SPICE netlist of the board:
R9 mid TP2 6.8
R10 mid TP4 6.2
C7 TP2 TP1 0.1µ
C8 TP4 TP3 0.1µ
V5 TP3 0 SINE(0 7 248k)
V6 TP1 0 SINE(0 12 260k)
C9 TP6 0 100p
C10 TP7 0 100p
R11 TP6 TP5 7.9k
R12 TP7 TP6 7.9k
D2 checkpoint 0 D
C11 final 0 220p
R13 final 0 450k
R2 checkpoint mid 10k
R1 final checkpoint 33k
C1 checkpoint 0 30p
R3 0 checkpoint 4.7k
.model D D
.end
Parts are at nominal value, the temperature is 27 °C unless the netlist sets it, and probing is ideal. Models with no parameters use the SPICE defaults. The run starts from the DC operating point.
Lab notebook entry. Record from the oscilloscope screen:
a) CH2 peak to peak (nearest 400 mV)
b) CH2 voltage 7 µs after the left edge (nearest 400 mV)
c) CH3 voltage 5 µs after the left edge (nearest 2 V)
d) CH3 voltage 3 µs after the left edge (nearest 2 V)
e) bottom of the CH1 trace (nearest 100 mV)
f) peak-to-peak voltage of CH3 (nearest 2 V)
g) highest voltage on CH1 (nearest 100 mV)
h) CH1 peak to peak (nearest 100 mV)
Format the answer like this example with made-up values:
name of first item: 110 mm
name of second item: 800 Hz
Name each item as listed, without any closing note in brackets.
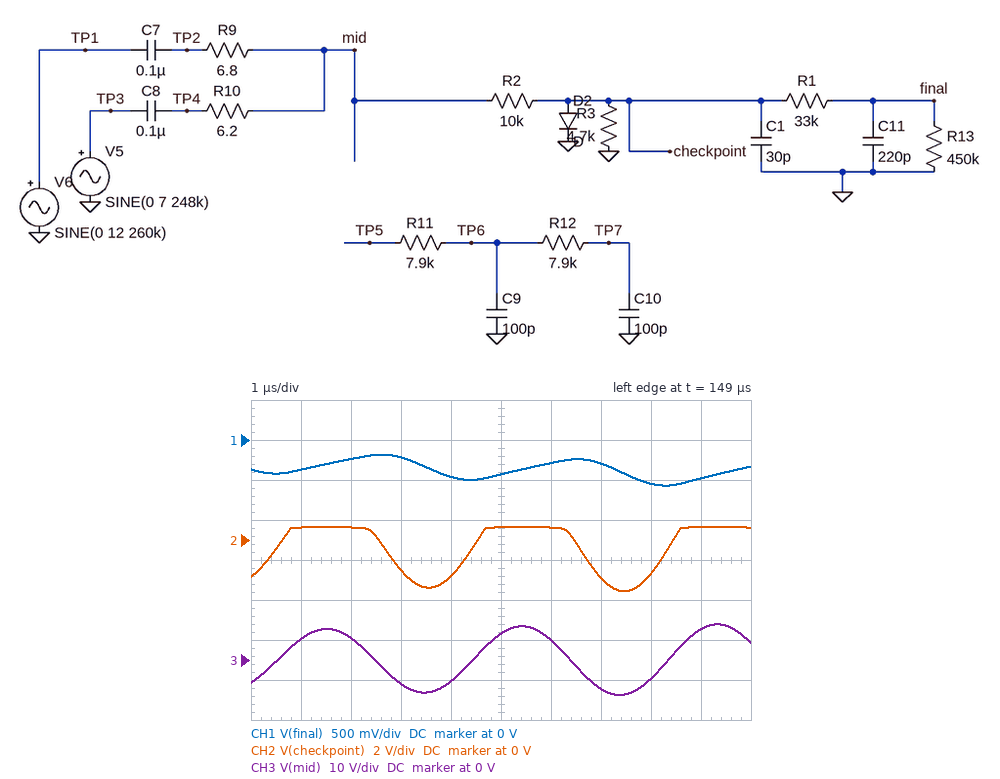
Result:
CH2 peak to peak: 3.2 V
CH2 voltage 7 µs after the left edge: -2.0 V
CH3 voltage 5 µs after the left edge: 6 V
CH3 voltage 3 µs after the left edge: -6 V
bottom of the CH1 trace: -600 mV
peak-to-peak voltage of CH3: 18 V
highest voltage on CH1: -200 mV
CH1 peak to peak: 400 mV
